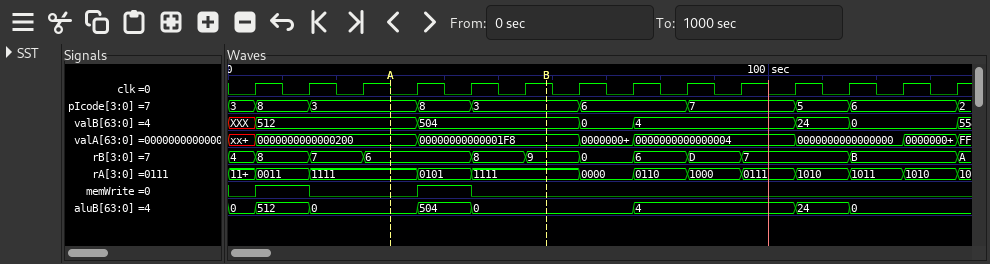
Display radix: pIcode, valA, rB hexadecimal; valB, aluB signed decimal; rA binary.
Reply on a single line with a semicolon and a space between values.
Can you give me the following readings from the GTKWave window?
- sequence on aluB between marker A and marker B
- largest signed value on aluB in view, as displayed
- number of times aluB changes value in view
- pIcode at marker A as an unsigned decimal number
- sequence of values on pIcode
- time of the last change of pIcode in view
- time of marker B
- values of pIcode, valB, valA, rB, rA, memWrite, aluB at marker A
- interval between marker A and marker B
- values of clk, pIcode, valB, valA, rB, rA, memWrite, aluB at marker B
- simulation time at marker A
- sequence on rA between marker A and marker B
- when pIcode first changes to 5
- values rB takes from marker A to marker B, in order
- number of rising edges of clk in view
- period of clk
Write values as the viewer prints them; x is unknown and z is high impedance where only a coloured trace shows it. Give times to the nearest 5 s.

0, 504, 0; 512; 7; 3; 3, 8, 3, 8, 3, 6, 7, 5, 6, 2; 135 s; 60 s; pIcode=3, valB=512, valA=0000000000000200, rB=6, rA=1111, memWrite=0, aluB=0; 30 s; clk=1, pIcode=3, valB=504, valA=00000000000001F8, rB=9, rA=1111, memWrite=0, aluB=0; 30 s; 1111, 0101, 1111; 105 s; 6, 8, 9; 14; 10 s
